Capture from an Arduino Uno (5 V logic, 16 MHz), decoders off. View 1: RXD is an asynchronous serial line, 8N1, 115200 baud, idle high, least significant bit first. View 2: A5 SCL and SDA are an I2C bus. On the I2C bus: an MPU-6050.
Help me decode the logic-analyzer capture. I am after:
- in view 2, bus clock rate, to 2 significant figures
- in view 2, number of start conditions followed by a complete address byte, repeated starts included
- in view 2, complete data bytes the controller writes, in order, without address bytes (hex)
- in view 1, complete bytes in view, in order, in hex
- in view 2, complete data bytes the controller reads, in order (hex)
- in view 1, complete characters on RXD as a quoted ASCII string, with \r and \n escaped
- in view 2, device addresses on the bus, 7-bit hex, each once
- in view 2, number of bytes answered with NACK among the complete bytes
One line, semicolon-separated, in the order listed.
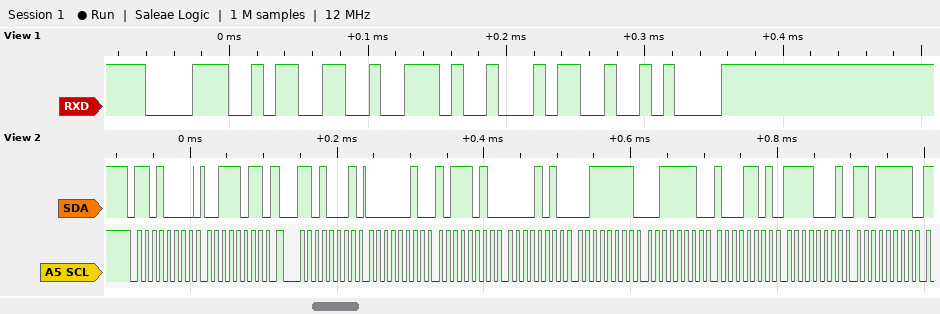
100 kHz; 2; 3B; 38 33 2E 34 0A; 02 BA 0A 3F 3E 8D F1 DF; "83.4\n"; 0x68; 0
